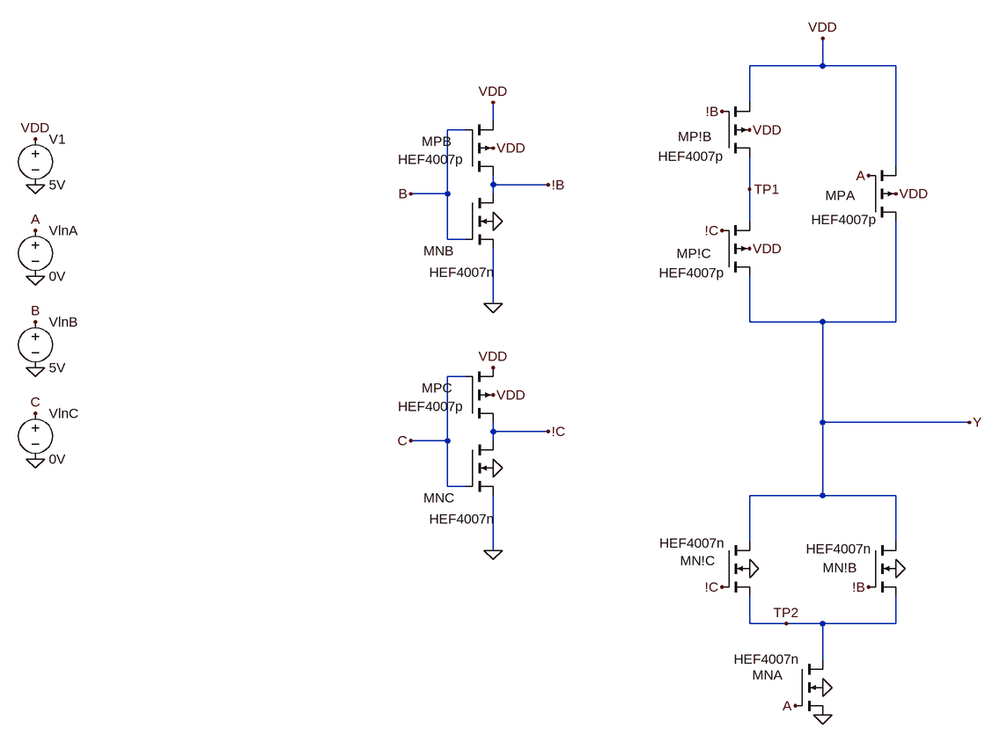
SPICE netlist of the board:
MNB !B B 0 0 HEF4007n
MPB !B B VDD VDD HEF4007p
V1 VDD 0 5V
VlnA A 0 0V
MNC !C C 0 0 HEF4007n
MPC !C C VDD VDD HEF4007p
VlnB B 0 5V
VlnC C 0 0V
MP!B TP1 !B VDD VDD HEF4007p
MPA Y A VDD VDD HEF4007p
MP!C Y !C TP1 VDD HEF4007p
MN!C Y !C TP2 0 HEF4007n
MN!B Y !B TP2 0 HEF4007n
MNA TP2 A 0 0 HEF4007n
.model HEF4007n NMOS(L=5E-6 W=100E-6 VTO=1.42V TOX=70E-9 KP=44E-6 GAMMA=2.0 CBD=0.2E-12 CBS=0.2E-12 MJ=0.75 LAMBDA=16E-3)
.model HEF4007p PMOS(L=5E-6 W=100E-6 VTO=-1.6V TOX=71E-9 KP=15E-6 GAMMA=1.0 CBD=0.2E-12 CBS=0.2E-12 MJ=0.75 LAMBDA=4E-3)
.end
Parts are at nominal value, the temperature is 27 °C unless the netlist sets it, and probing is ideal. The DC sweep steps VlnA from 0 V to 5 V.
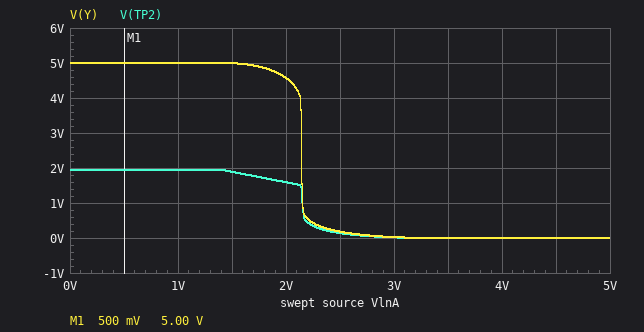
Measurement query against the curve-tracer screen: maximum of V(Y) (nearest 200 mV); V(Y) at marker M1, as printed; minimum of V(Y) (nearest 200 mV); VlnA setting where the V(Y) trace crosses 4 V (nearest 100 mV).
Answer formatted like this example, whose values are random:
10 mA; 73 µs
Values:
5.0 V; 5.00 V; 0 V; 2.1 V
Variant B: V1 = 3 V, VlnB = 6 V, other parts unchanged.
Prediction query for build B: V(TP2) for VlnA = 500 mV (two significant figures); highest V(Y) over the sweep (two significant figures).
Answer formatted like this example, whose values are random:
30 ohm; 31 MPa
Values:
780 mV; 3.0 V
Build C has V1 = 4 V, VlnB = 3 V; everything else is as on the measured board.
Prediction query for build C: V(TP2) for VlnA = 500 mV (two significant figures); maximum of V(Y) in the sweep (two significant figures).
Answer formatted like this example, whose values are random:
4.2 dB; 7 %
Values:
1.3 V; 4.0 V
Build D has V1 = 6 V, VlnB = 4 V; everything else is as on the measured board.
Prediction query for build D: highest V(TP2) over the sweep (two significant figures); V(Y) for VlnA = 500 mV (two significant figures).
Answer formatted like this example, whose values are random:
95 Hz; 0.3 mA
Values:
2.6 V; 6.0 V
